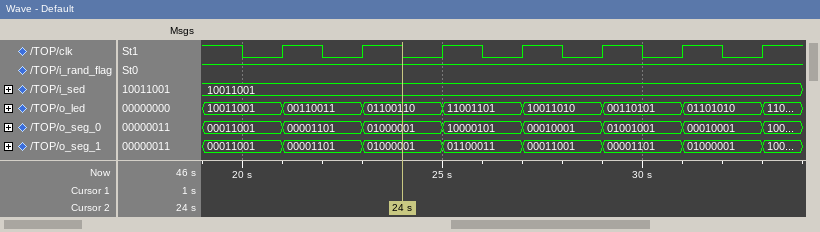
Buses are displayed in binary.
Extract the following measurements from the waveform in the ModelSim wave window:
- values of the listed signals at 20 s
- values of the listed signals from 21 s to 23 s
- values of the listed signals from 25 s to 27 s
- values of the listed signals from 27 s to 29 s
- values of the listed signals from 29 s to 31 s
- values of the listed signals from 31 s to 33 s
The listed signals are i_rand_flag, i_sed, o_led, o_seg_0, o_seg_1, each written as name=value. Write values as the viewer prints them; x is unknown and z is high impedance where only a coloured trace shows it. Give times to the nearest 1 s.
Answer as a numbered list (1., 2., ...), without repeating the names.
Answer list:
1. i_rand_flag=1, i_sed=10011001, o_led=10011001, o_seg_0=00011001, o_seg_1=00011001
2. i_rand_flag=1, i_sed=10011001, o_led=00110011, o_seg_0=00001101, o_seg_1=00001101
3. i_rand_flag=1, i_sed=10011001, o_led=11001101, o_seg_0=10000101, o_seg_1=01100011
4. i_rand_flag=1, i_sed=10011001, o_led=10011010, o_seg_0=00010001, o_seg_1=00011001
5. i_rand_flag=1, i_sed=10011001, o_led=00110101, o_seg_0=01001001, o_seg_1=00001101
6. i_rand_flag=1, i_sed=10011001, o_led=01101010, o_seg_0=00010001, o_seg_1=01000001
